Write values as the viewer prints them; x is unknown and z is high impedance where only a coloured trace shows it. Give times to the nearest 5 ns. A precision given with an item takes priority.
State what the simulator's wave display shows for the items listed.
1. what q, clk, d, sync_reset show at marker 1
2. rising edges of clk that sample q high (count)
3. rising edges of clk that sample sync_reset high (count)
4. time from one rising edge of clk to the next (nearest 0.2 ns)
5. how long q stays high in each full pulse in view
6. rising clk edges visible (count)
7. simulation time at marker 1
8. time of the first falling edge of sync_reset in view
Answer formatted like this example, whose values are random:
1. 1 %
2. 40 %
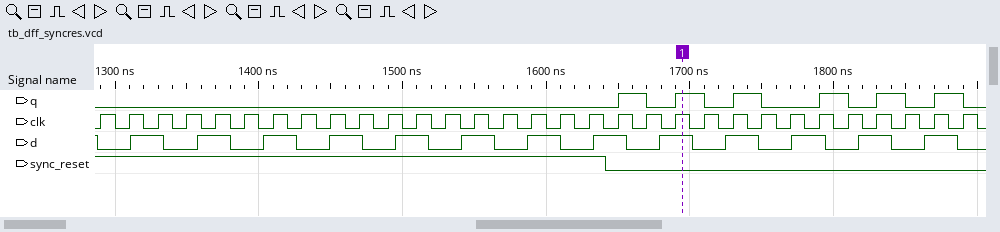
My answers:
1. q=1, clk=1, d=1, sync_reset=0
2. 6
3. 18
4. 20 ns
5. 20 ns, 20 ns, 20 ns, 20 ns, 20 ns, 20 ns
6. 31
7. 1695 ns
8. 1640 ns
